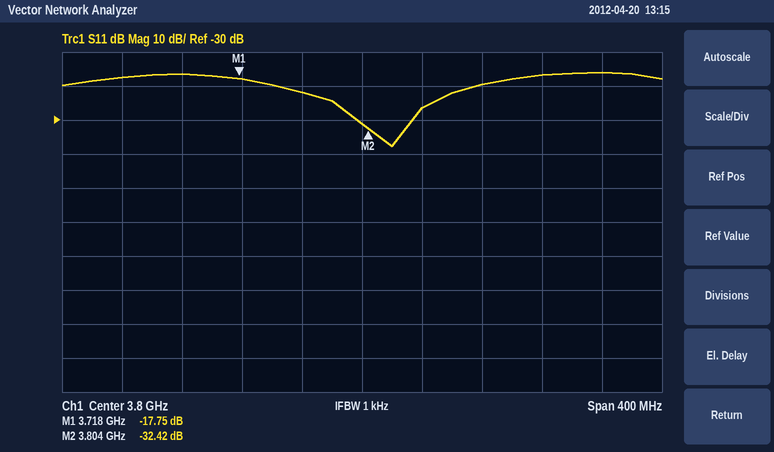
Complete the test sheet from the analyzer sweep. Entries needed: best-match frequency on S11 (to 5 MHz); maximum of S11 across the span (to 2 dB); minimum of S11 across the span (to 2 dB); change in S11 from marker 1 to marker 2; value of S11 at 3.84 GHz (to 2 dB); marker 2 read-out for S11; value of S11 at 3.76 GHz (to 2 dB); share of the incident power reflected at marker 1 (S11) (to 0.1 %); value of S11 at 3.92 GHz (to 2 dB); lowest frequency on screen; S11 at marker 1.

3.820 GHz
-16 dB
-38 dB
-14.67 dB
-26 dB
-32.42 dB
-22 dB
1.7 %
-16 dB
3.6 GHz
-17.75 dB
